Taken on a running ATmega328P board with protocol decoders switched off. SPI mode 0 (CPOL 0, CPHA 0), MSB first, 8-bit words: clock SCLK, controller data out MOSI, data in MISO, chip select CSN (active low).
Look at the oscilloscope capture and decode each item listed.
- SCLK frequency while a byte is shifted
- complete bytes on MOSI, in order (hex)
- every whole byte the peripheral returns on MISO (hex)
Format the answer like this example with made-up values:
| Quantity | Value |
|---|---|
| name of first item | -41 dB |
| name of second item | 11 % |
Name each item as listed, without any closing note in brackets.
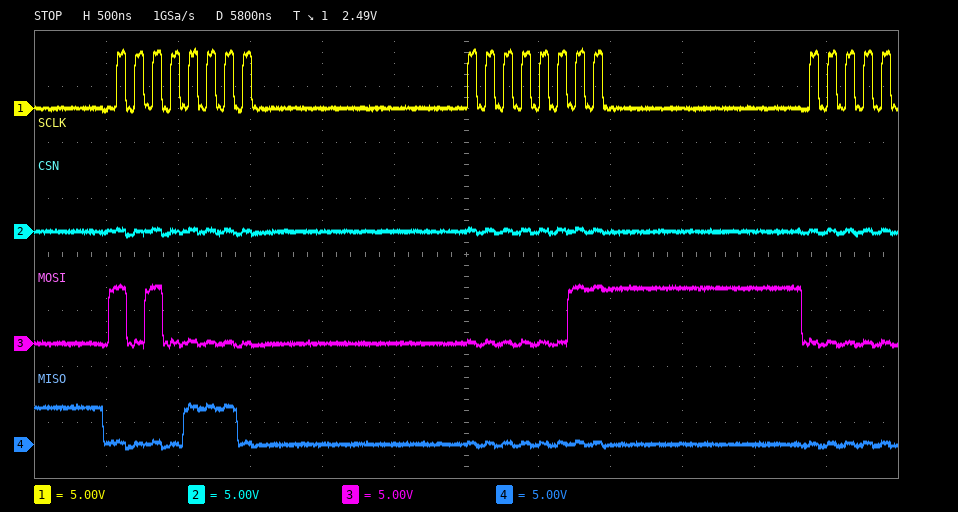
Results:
| Quantity | Value |
|---|---|
| SCLK frequency while a byte is shifted | 8 MHz |
| complete bytes on MOSI, in order | 0xA0 0x03 |
| every whole byte the peripheral returns on MISO | 0x0E 0x00 |
